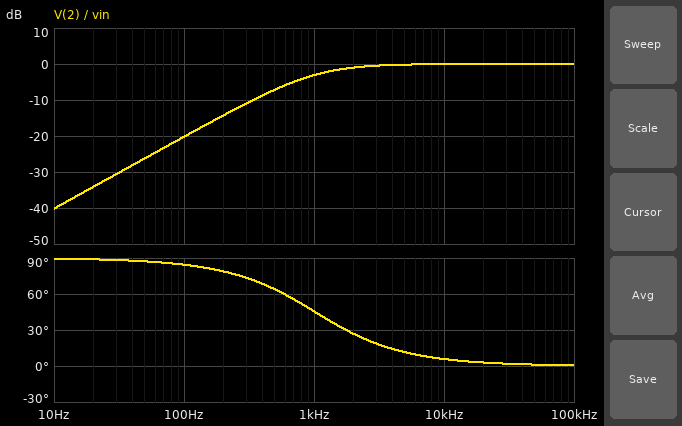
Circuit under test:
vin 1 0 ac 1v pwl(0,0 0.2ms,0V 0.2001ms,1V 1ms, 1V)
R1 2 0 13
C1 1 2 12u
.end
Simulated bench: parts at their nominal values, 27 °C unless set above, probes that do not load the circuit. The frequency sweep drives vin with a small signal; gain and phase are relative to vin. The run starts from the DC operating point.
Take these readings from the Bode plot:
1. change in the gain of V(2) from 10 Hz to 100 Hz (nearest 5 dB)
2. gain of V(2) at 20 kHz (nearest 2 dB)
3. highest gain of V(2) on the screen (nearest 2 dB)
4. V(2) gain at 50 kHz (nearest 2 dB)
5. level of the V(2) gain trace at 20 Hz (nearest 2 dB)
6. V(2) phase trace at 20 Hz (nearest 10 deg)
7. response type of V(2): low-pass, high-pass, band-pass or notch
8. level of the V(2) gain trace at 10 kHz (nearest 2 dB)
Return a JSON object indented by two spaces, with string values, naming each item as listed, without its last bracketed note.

{
  "change in the gain of V(2) from 10 Hz to 100 Hz": "20 dB",
  "gain of V(2) at 20 kHz": "0 dB",
  "highest gain of V(2) on the screen": "0 dB",
  "V(2) gain at 50 kHz": "0 dB",
  "level of the V(2) gain trace at 20 Hz": "-34 dB",
  "V(2) phase trace at 20 Hz": "90 deg",
  "response type of V(2): low-pass, high-pass, band-pass or notch": "high-pass",
  "level of the V(2) gain trace at 10 kHz": "0 dB"
}
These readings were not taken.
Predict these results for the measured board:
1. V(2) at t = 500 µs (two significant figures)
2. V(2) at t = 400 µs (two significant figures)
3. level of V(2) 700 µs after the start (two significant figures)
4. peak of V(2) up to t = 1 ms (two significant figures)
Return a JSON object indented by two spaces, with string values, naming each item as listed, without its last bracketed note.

{
  "V(2) at t = 500 µs": "150 mV",
  "V(2) at t = 400 µs": "280 mV",
  "level of V(2) 700 µs after the start": "41 mV",
  "peak of V(2) up to t = 1 ms": "1.0 V"
}
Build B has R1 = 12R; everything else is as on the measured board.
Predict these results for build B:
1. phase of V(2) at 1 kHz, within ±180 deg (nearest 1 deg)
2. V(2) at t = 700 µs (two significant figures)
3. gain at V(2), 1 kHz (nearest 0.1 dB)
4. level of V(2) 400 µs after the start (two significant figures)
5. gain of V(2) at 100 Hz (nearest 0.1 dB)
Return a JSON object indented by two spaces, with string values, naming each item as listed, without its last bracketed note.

{
  "phase of V(2) at 1 kHz, within ±180 deg": "48 deg",
  "V(2) at t = 700 µs": "31 mV",
  "gain at V(2), 1 kHz": "-3.5 dB",
  "level of V(2) 400 µs after the start": "250 mV",
  "gain of V(2) at 100 Hz": "-20.9 dB"
}
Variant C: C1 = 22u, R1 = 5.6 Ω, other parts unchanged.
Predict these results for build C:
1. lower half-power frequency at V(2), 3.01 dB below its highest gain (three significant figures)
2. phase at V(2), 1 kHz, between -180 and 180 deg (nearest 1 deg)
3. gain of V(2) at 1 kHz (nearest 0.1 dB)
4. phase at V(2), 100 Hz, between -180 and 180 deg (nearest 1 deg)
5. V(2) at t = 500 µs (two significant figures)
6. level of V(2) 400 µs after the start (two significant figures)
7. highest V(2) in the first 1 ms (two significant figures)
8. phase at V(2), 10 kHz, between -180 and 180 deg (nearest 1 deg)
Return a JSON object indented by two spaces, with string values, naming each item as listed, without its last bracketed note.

{
  "lower half-power frequency at V(2), 3.01 dB below its highest gain": "1.29 kHz",
  "phase at V(2), 1 kHz, between -180 and 180 deg": "52 deg",
  "gain of V(2) at 1 kHz": "-4.3 dB",
  "phase at V(2), 100 Hz, between -180 and 180 deg": "86 deg",
  "V(2) at t = 500 µs": "88 mV",
  "level of V(2) 400 µs after the start": "200 mV",
  "highest V(2) in the first 1 ms": "1.0 V",
  "phase at V(2), 10 kHz, between -180 and 180 deg": "7 deg"
}
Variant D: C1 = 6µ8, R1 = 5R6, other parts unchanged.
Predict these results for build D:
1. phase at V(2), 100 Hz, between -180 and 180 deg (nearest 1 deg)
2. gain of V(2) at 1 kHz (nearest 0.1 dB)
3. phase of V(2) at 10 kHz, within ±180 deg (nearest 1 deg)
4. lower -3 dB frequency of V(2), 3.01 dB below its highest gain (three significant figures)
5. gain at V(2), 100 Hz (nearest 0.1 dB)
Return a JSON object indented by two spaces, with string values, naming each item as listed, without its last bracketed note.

{
  "phase at V(2), 100 Hz, between -180 and 180 deg": "89 deg",
  "gain of V(2) at 1 kHz": "-12.7 dB",
  "phase of V(2) at 10 kHz, within ±180 deg": "23 deg",
  "lower -3 dB frequency of V(2), 3.01 dB below its highest gain": "4.18 kHz",
  "gain at V(2), 100 Hz": "-32.4 dB"
}
